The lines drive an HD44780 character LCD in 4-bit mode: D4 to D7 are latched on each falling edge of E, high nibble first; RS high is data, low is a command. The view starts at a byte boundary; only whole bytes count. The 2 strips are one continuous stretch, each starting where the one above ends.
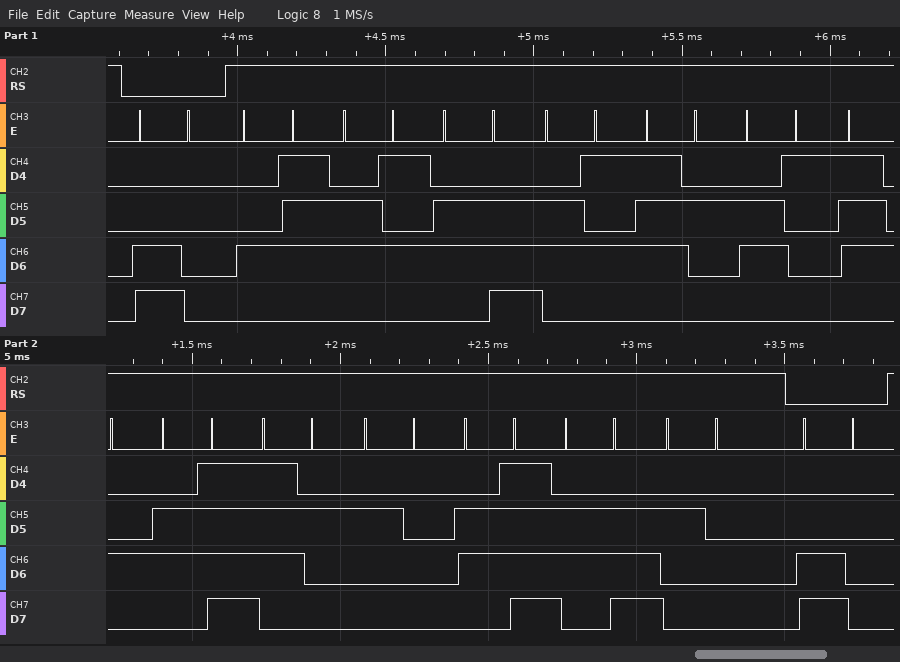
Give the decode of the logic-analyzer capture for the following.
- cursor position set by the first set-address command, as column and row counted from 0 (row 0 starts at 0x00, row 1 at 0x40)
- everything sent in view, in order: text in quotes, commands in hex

column 0, row 1
0xC0 "Generator on " 0xC0
